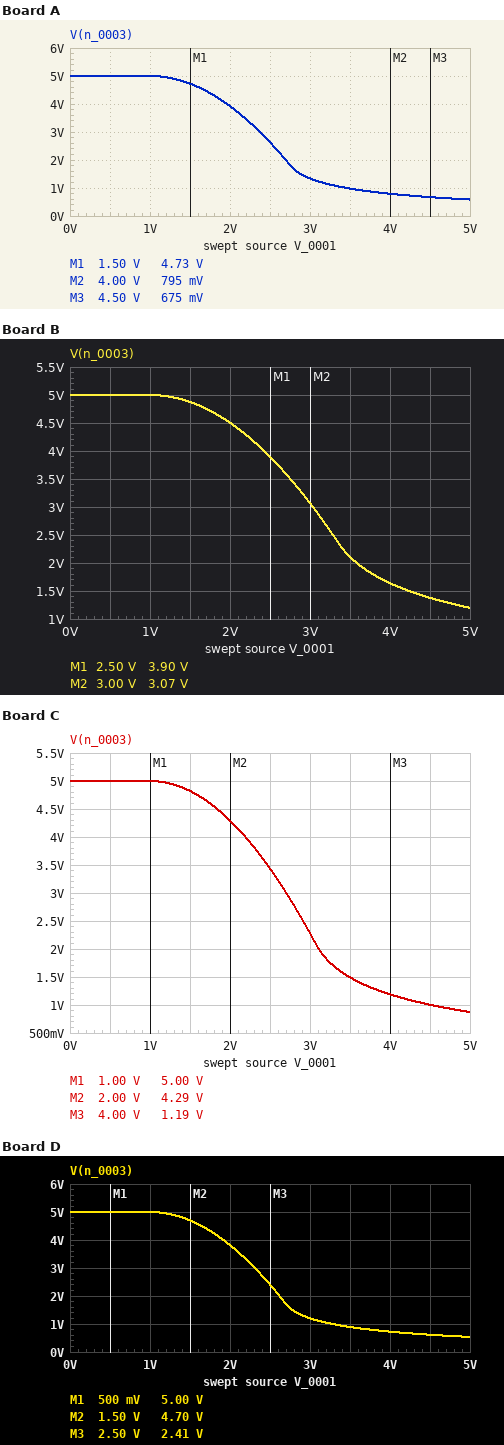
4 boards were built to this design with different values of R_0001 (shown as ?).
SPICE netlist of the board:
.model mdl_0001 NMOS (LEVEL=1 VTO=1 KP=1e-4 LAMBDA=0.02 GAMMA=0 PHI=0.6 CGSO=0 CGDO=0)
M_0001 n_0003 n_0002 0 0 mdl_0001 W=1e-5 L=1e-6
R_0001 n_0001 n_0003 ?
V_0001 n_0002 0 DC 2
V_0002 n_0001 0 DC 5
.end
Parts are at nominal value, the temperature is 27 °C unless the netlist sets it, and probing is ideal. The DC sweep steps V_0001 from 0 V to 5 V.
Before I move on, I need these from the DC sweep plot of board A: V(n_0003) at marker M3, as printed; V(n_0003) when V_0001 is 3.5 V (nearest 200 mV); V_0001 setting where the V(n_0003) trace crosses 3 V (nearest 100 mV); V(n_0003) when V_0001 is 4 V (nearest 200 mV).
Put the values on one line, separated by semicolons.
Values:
675 mV; 1.0 V; 2.4 V; 800 mV
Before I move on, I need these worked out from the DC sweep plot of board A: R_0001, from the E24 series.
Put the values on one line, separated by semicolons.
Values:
2 kΩ
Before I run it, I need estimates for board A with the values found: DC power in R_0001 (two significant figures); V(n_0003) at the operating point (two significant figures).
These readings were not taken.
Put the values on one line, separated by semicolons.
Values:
580 µW; 3.9 V
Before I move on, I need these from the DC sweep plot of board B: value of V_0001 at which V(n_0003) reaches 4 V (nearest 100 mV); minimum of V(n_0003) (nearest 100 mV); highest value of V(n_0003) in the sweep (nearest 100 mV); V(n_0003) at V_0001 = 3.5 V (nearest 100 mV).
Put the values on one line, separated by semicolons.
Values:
2.4 V; 1.2 V; 5.0 V; 2.1 V
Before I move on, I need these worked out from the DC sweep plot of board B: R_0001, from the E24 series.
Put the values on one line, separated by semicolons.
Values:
910 Ω
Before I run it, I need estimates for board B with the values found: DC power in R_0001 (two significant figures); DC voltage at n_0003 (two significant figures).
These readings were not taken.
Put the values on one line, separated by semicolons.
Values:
270 µW; 4.5 V
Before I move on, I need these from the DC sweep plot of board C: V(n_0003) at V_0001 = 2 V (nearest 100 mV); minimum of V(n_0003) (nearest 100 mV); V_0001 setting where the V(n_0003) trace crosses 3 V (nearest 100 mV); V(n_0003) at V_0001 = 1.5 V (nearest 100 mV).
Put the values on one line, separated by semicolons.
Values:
4.3 V; 900 mV; 2.7 V; 4.8 V
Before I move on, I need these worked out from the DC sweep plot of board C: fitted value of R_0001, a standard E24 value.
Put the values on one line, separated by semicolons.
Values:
1.3 kΩ
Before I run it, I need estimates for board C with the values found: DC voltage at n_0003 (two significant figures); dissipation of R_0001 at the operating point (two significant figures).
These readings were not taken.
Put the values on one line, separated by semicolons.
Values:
4.3 V; 380 µW
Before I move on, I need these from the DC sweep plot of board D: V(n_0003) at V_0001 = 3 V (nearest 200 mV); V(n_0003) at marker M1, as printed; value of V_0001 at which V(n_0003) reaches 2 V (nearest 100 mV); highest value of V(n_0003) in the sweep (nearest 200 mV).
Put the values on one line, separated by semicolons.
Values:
1.2 V; 5.00 V; 2.6 V; 5.0 V
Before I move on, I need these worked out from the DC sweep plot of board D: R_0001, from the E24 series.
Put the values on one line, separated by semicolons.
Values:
2.2 kΩ
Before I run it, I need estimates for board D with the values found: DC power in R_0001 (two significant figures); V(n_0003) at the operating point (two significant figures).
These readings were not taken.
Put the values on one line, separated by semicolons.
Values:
640 µW; 3.8 V
